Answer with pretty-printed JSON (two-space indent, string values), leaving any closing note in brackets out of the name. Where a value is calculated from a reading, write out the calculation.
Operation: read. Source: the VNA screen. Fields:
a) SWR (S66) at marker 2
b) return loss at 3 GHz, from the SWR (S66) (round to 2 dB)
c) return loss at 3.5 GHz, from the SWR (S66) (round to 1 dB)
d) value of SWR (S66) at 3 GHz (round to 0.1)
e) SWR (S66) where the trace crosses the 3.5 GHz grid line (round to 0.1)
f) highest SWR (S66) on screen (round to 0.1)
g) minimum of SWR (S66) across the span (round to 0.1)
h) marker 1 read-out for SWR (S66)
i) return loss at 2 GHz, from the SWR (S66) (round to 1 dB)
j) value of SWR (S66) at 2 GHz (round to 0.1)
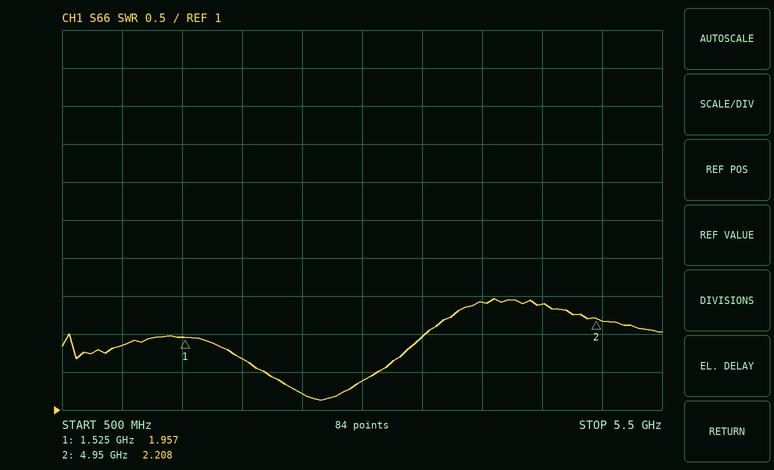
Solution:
{
  "SWR (S66) at marker 2": "2.208",
  "return loss at 3 GHz, from the SWR (S66)": "−20 log10((1.4 − 1)/(1.4 + 1)) ≈ 16 dB",
  "return loss at 3.5 GHz, from the SWR (S66)": "−20 log10((2 − 1)/(2 + 1)) ≈ 10 dB",
  "value of SWR (S66) at 3 GHz": "1.4",
  "SWR (S66) where the trace crosses the 3.5 GHz grid line": "2.0",
  "highest SWR (S66) on screen": "2.5",
  "minimum of SWR (S66) across the span": "1.1",
  "marker 1 read-out for SWR": "1.957",
  "return loss at 2 GHz, from the SWR (S66)": "−20 log10((1.7 − 1)/(1.7 + 1)) ≈ 12 dB",
  "value of SWR (S66) at 2 GHz": "1.7"
}
